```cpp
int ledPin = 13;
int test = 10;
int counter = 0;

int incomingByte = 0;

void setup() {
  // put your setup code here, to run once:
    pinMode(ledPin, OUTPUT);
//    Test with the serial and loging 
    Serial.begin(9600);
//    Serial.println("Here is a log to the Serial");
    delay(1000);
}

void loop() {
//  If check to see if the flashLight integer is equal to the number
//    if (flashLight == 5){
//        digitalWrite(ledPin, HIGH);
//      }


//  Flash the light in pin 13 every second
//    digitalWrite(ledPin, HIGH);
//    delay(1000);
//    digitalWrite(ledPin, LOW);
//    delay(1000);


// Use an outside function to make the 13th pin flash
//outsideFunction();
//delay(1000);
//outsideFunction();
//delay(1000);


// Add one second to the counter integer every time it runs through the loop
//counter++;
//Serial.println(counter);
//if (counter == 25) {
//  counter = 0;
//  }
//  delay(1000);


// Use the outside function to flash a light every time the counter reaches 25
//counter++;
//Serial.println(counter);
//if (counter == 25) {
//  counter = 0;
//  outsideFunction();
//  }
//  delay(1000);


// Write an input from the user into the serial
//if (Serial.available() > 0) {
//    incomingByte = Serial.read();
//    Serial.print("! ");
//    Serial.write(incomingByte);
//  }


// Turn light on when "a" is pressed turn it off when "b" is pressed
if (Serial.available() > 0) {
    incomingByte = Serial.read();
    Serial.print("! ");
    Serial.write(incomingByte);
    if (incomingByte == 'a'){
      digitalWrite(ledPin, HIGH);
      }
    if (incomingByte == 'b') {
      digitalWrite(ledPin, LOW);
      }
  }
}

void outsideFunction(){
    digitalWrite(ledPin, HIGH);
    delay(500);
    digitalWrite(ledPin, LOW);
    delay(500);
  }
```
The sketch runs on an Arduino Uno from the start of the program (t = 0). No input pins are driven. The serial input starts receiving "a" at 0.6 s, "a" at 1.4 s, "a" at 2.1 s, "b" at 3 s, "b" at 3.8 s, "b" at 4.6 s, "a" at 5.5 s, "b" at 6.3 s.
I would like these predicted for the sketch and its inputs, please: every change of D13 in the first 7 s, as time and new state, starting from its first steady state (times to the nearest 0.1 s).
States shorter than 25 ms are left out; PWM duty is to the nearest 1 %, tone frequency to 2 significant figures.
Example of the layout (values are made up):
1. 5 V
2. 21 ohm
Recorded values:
1. 0 s low; 1 s high; 3 s low; 5.5 s high; 6.3 s low
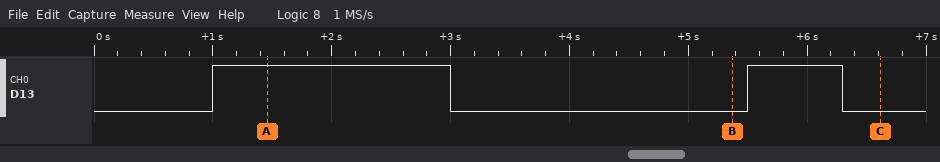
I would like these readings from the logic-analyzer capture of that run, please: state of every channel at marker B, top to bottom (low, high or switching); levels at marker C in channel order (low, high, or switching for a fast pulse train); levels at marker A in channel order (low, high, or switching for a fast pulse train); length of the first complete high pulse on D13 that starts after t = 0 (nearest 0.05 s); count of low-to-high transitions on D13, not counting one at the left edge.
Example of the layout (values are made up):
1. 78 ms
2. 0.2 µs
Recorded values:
1. D13 low
2. D13 low
3. D13 high
4. 2.00 s
5. 2
